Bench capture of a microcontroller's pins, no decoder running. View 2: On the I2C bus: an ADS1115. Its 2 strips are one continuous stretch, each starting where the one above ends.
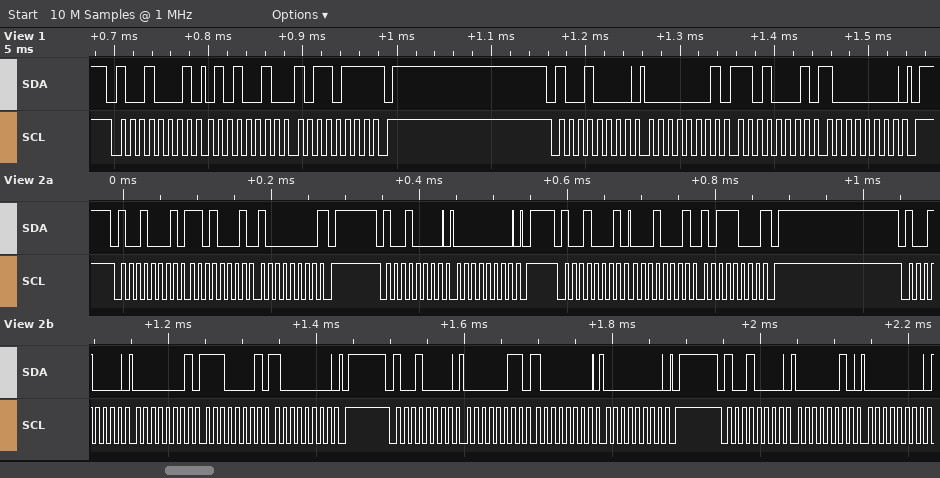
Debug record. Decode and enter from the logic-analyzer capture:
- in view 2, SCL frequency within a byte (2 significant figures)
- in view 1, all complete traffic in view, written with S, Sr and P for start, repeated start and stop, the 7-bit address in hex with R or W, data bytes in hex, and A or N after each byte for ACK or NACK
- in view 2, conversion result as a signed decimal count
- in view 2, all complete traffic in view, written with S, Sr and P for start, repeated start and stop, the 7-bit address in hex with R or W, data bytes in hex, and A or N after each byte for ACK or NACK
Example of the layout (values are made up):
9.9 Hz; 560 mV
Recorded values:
100 kHz; S 48R A 52 A B7 N P S 48W A 01 A D1 A 80 A P; 4536; S 48R A D1 A 80 N P S 48W A 00 A P S 48R A 11 A B8 N P S 48W A 01 A E1 A 80 A P S 48W A 03 A 80 A 00 A P S 48W A 02 A 00 A
